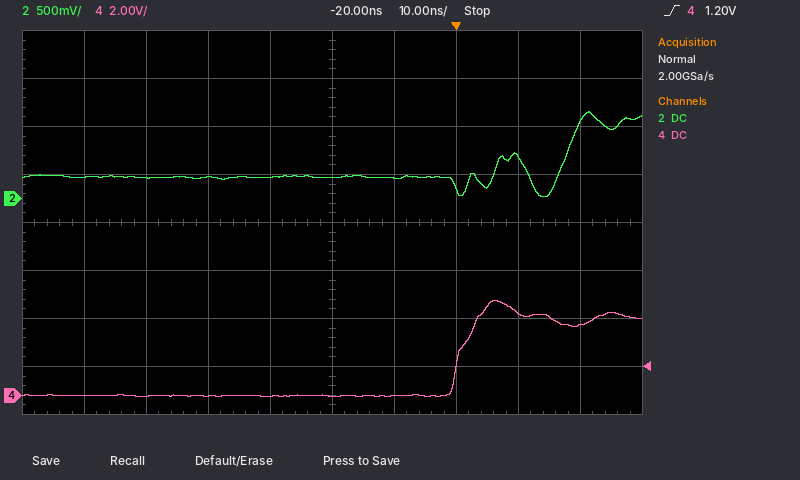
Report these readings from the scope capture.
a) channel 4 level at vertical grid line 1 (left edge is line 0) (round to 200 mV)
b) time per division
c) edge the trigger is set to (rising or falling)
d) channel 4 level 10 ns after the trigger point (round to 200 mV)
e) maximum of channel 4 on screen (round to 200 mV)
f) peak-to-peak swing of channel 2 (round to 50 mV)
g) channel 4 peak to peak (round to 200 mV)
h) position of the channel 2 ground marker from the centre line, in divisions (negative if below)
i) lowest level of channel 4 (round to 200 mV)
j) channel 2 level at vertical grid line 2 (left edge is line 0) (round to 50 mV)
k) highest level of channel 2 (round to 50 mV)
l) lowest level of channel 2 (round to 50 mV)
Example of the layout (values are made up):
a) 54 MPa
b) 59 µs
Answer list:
a) 0.0 V
b) 10 ns
c) rising
d) 3.4 V
e) 4.0 V
f) 900 mV
g) 4.0 V
h) +0.5 div
i) 0.0 V
j) 200 mV
k) 900 mV
l) 0 mV
